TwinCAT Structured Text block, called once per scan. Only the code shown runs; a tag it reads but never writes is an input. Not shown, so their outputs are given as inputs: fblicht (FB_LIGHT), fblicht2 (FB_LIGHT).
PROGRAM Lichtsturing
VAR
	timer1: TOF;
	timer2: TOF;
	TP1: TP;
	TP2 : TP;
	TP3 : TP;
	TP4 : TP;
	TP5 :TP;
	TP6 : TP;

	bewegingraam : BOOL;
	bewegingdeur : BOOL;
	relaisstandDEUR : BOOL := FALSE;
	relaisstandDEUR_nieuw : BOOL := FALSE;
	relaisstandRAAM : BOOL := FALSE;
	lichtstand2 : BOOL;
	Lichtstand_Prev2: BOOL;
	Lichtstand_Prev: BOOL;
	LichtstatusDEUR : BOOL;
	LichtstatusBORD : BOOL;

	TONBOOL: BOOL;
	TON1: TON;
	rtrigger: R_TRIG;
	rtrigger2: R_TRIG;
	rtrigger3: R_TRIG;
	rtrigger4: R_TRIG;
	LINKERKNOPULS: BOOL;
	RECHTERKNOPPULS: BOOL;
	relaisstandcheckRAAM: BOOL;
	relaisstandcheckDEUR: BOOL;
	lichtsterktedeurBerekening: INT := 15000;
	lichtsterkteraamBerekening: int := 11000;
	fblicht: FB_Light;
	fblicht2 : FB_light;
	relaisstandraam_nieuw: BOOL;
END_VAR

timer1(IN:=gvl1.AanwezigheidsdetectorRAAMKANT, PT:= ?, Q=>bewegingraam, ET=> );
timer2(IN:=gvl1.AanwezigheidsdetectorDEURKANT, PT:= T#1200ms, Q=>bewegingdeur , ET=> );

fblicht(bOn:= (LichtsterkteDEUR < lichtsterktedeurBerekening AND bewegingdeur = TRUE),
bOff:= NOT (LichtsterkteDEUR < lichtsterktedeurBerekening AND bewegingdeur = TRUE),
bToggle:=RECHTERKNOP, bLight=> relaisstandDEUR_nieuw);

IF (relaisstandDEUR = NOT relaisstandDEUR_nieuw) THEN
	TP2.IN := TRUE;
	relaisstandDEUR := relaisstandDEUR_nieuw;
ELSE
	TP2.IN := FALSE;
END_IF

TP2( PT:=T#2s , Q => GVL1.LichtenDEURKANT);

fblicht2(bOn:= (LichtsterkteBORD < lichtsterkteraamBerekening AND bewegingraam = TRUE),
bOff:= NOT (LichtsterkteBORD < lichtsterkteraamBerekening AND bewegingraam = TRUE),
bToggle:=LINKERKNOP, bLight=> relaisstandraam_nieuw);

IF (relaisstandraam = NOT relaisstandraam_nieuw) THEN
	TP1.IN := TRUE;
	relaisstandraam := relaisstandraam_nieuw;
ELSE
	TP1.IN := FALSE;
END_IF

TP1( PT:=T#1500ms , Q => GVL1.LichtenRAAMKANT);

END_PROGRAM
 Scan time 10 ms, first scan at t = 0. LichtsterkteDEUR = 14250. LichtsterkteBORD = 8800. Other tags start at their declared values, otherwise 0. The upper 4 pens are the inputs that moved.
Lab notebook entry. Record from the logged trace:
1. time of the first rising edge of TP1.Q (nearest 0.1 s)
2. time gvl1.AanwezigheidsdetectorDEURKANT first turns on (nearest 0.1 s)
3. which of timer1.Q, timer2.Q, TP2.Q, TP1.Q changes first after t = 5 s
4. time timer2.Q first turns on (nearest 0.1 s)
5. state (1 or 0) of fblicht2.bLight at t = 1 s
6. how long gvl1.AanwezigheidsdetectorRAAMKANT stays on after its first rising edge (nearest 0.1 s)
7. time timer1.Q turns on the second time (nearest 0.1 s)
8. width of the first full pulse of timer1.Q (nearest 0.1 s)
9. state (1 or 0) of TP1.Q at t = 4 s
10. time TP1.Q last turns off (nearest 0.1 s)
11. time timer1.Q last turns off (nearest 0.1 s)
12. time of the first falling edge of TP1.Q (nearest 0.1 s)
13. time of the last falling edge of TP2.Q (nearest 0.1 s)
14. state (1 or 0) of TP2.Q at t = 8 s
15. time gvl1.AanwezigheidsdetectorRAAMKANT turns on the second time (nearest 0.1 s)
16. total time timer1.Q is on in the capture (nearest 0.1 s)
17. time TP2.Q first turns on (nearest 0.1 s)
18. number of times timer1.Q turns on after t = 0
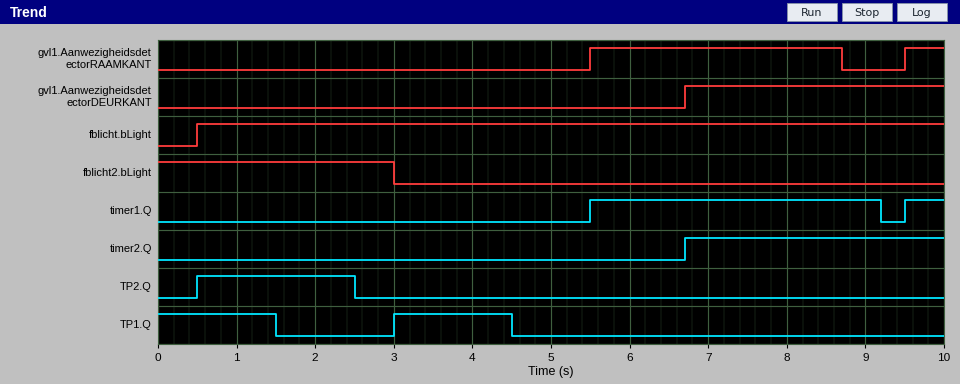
3.0 s
6.7 s
timer1.Q
6.7 s
1
3.2 s
9.5 s
3.7 s
1
4.5 s
9.2 s
1.5 s
2.5 s
0
9.5 s
4.2 s
0.5 s
2
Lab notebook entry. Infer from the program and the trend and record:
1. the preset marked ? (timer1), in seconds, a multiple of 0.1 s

0.5 s
